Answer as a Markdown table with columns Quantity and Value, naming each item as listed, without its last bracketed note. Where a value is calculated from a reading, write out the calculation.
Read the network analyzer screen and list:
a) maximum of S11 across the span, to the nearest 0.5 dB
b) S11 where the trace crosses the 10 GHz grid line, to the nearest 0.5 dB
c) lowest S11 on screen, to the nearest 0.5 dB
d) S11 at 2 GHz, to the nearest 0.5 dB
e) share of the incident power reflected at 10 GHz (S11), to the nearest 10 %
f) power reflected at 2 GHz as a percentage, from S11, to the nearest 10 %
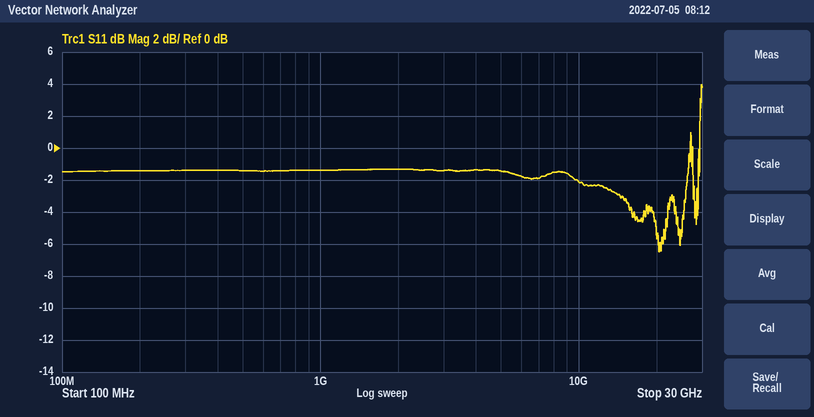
| Quantity | Value |
|---|---|
| maximum of S11 across the span, to the nearest 0.5 dB | 4.0 dB |
| S11 where the trace crosses the 10 GHz grid line, to the nearest 0.5 dB | -2.0 dB |
| lowest S11 on screen, to the nearest 0.5 dB | -6.5 dB |
| S11 at 2 GHz, to the nearest 0.5 dB | -1.5 dB |
| share of the incident power reflected at 10 GHz (S11), to the nearest 10 % | 10^(-2/10) ≈ 63.1 %, so 60 % to the nearest 10 % |
| power reflected at 2 GHz as a percentage, from S11, to the nearest 10 % | 10^(-1.5/10) ≈ 70.8 %, so 70 % to the nearest 10 % |
